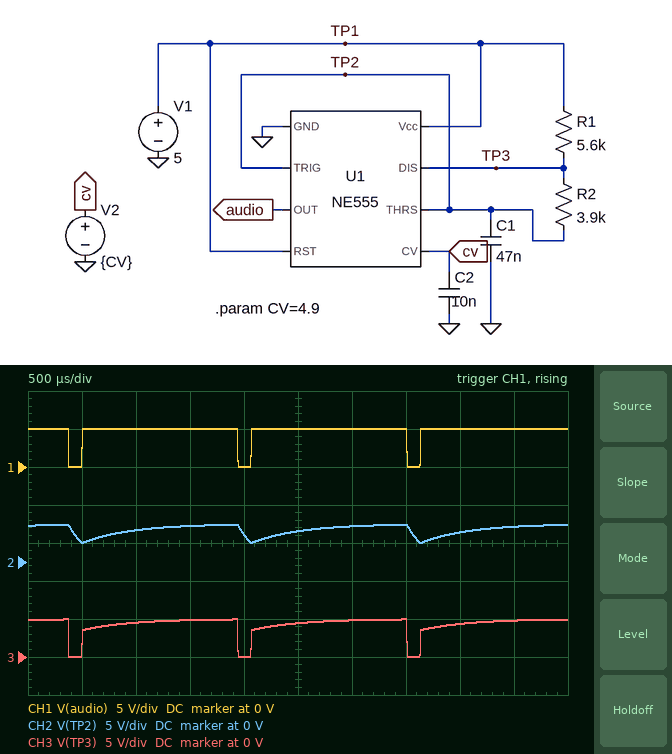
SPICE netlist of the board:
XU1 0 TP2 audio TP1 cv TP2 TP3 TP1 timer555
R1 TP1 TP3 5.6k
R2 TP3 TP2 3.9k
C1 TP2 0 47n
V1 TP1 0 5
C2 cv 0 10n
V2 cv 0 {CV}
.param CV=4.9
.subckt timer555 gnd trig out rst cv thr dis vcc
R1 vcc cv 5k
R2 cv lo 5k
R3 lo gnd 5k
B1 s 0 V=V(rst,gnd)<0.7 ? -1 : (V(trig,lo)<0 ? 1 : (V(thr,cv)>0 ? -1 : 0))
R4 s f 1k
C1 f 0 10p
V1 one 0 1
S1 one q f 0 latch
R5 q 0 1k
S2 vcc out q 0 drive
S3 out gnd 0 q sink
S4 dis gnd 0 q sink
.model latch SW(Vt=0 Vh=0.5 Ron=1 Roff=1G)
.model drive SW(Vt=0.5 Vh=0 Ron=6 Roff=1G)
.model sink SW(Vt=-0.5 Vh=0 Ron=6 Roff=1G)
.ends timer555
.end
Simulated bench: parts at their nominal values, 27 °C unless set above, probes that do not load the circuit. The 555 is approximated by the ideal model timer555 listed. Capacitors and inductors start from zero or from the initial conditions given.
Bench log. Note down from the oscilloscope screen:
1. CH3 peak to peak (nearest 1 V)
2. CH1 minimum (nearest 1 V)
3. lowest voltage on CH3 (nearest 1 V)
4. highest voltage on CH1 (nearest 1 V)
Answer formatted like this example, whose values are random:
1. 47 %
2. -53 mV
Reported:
1. 5 V
2. 0 V
3. 0 V
4. 5 V
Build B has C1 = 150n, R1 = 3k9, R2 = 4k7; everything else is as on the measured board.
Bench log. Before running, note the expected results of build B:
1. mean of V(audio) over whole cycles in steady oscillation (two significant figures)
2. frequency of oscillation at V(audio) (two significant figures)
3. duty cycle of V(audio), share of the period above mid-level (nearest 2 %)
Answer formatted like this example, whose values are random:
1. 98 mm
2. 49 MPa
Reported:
1. 4.5 V
2. 210 Hz
3. 90 %
